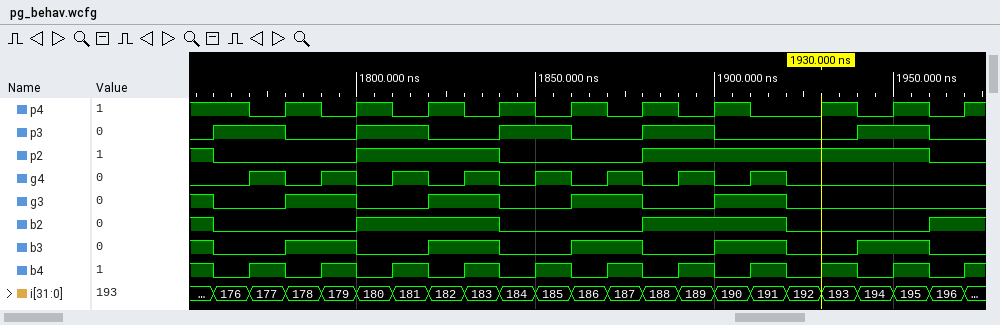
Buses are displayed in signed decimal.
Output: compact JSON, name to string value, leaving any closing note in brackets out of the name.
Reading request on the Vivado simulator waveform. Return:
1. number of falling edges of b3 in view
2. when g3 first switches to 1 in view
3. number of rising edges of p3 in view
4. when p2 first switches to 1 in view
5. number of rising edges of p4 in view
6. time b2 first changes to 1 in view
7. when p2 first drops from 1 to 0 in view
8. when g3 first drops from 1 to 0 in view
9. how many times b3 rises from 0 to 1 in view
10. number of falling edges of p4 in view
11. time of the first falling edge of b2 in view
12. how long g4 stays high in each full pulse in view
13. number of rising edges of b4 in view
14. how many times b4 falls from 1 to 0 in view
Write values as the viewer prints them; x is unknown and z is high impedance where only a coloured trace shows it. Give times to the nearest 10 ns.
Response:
{"number of falling edges of b3 in view": "6", "when g3 first switches to 1 in view": "1780 ns", "number of rising edges of p3 in view": "5", "when p2 first switches to 1 in view": "1800 ns", "number of rising edges of p4 in view": "10", "time b2 first changes to 1 in view": "1800 ns", "when p2 first drops from 1 to 0 in view": "1760 ns", "when g3 first drops from 1 to 0 in view": "1760 ns", "how many times b3 rises from 0 to 1 in view": "5", "number of falling edges of p4 in view": "10", "time of the first falling edge of b2 in view": "1760 ns", "how long g4 stays high in each full pulse in view": "10 ns, 10 ns, 10 ns, 10 ns, 10 ns, 10 ns, 10 ns, 10 ns", "number of rising edges of b4 in view": "11", "how many times b4 falls from 1 to 0 in view": "11"}
